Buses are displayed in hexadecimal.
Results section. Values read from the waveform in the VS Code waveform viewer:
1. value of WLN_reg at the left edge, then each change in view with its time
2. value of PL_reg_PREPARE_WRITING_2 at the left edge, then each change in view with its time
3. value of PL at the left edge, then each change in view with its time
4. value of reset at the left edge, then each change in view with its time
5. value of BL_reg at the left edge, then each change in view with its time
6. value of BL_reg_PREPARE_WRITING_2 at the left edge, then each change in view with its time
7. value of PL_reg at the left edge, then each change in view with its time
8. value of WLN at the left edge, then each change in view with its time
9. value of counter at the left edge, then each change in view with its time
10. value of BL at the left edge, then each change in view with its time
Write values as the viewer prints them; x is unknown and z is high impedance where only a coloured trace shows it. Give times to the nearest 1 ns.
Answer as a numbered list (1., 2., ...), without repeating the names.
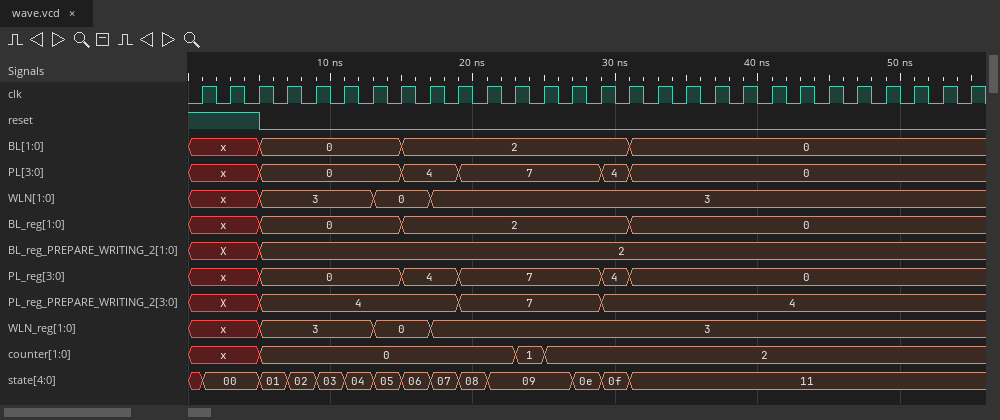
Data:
1. x, 3 at 5 ns, 0 at 13 ns, 3 at 17 ns
2. X, 4 at 5 ns, 7 at 19 ns, 4 at 29 ns
3. x, 0 at 5 ns, 4 at 15 ns, 7 at 19 ns, 4 at 29 ns, 0 at 31 ns
4. 1, 0 at 5 ns
5. x, 0 at 5 ns, 2 at 15 ns, 0 at 31 ns
6. X, 2 at 5 ns
7. x, 0 at 5 ns, 4 at 15 ns, 7 at 19 ns, 4 at 29 ns, 0 at 31 ns
8. x, 3 at 5 ns, 0 at 13 ns, 3 at 17 ns
9. x, 0 at 5 ns, 1 at 23 ns, 2 at 25 ns
10. x, 0 at 5 ns, 2 at 15 ns, 0 at 31 ns
